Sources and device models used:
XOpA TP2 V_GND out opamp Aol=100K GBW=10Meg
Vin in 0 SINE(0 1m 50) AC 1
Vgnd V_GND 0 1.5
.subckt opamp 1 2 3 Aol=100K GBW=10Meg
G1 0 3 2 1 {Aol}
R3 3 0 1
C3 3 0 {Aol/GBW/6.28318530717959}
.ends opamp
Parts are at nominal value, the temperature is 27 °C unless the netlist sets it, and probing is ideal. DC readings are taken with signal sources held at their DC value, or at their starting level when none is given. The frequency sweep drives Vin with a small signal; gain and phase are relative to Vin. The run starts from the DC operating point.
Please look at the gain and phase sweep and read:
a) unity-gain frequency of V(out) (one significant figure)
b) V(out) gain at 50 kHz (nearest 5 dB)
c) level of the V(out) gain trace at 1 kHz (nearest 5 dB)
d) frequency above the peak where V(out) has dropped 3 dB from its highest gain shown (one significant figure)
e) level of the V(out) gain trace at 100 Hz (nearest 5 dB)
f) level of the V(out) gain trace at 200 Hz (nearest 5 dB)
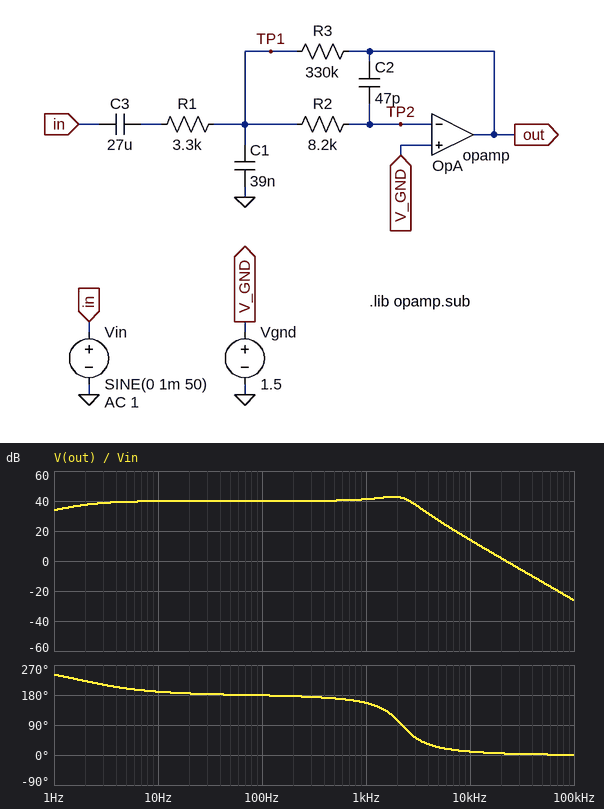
20 kHz
-15 dB
40 dB
3 kHz
40 dB
40 dB
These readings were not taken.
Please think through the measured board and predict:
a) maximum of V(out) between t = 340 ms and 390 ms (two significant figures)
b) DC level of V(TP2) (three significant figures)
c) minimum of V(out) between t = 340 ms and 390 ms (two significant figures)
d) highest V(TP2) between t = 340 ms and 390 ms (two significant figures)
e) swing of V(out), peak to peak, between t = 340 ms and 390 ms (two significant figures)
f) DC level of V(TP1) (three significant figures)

1.6 V
1.50 V
1.4 V
1.5 V
200 mV
1.50 V
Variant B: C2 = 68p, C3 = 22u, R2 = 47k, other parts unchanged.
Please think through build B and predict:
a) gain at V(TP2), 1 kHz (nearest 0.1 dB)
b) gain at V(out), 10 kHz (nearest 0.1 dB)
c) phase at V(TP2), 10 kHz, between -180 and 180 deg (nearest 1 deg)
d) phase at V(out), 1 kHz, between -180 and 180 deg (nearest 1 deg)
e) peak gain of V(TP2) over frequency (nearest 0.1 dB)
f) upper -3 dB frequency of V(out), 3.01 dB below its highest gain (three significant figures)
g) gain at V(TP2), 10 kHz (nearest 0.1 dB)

-47.1 dB
-4.3 dB
-83 deg
74 deg
-46.7 dB
628 Hz
-64.3 dB
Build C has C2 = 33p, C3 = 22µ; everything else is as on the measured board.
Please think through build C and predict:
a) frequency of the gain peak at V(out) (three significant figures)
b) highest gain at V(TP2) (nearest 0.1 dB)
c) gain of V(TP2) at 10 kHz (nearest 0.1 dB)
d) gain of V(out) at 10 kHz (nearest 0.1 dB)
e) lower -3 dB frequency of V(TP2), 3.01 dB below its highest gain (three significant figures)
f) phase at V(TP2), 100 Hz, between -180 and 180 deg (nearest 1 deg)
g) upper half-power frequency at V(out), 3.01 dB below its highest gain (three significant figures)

2.32 kHz
-28.0 dB
-42.8 dB
17.2 dB
1.90 kHz
45 deg
3.11 kHz
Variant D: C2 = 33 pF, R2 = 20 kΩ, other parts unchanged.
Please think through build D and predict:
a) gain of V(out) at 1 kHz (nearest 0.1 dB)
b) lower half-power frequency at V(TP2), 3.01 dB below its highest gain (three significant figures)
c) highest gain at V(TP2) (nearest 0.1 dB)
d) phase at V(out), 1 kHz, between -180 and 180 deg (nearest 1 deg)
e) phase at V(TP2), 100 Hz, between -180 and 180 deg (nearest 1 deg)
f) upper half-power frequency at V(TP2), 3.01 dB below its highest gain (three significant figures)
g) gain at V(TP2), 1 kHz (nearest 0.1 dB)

41.7 dB
1.13 kHz
-33.9 dB
143 deg
43 deg
2.58 kHz
-38.3 dB
